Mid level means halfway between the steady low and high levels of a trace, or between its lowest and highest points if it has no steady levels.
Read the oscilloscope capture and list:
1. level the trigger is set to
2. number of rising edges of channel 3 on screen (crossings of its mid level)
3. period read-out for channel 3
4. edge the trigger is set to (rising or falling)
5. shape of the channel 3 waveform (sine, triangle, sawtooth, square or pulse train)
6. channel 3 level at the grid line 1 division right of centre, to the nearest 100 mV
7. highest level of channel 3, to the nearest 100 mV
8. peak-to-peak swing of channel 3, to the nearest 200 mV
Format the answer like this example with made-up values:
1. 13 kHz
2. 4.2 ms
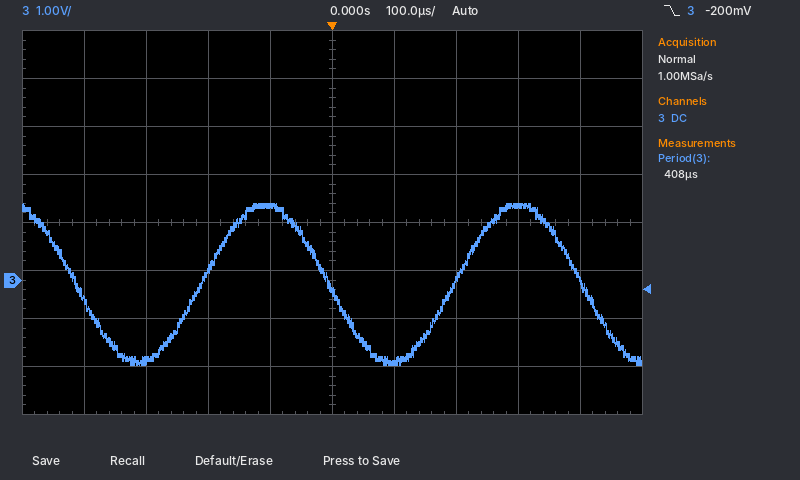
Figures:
1. -200 mV
2. 2
3. 408 µs
4. falling
5. sine
6. -1.7 V
7. 1.6 V
8. 3.4 V
